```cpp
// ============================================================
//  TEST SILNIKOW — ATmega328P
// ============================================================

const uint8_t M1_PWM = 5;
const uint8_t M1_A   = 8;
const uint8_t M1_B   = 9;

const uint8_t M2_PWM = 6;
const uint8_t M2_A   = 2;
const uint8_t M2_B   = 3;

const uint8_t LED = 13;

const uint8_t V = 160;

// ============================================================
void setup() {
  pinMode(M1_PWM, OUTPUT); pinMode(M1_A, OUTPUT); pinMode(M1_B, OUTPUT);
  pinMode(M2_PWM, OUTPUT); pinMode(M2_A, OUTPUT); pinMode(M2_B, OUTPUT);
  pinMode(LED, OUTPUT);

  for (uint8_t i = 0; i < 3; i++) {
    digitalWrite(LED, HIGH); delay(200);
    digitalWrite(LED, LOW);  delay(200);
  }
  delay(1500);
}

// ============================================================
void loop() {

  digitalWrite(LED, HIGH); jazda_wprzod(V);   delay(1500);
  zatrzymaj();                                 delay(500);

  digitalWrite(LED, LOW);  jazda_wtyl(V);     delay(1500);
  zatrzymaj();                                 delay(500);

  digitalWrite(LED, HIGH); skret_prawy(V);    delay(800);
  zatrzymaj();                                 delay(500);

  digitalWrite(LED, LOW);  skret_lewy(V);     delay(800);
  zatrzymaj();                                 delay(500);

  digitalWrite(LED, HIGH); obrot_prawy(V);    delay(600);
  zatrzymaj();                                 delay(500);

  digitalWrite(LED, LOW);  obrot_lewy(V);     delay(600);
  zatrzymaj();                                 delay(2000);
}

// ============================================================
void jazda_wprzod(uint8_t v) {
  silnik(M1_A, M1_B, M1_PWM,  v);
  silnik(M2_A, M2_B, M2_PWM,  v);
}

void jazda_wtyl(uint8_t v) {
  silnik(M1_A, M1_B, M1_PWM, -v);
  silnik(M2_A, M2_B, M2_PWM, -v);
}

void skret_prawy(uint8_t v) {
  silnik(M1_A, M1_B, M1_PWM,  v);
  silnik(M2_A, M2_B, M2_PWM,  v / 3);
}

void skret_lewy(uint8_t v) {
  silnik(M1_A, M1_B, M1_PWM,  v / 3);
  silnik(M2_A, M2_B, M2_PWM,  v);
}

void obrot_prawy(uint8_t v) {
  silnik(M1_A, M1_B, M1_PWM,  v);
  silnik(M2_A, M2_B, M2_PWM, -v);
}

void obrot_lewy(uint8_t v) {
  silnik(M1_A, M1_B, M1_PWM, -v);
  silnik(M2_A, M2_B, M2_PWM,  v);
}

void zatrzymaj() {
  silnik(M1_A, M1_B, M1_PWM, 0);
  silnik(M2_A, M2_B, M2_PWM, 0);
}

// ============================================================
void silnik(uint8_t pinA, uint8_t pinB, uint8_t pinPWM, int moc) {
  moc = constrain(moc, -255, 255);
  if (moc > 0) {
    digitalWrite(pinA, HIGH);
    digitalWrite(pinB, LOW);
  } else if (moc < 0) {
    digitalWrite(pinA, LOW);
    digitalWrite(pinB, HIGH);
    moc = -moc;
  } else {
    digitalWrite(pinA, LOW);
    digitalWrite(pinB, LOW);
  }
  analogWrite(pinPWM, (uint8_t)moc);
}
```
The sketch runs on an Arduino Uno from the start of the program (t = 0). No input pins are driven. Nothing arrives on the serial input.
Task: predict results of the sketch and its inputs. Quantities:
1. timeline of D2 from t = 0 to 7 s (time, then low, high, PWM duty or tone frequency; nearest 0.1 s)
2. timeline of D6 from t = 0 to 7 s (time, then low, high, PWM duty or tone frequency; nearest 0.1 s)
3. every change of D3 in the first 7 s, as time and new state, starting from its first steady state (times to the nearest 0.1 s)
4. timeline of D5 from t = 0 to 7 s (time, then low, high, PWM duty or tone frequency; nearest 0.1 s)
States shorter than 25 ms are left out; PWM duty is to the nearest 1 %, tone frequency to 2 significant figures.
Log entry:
0 s low; 2.7 s high; 4.2 s low; 6.7 s high
0 s low; 2.7 s PWM 63 %; 4.2 s low; 4.7 s PWM 63 %; 6.2 s low; 6.7 s PWM 21 %
0 s low; 4.7 s high; 6.2 s low
0 s low; 2.7 s PWM 63 %; 4.2 s low; 4.7 s PWM 63 %; 6.2 s low; 6.7 s PWM 63 %
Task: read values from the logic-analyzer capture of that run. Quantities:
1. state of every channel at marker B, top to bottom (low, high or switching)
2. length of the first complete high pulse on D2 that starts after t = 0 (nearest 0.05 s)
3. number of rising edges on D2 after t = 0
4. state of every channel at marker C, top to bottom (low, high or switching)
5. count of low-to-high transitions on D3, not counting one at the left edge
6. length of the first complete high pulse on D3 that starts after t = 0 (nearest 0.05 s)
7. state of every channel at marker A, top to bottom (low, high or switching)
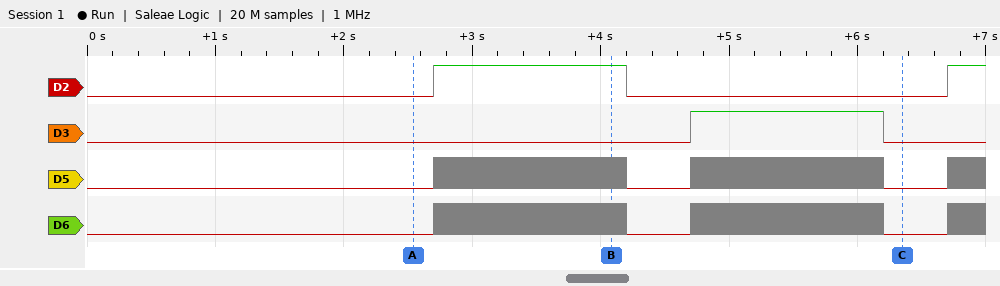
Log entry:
D2 high, D3 low, D5 switching, D6 switching
1.50 s
2
D2 low, D3 low, D5 low, D6 low
1
1.50 s
D2 low, D3 low, D5 low, D6 low
